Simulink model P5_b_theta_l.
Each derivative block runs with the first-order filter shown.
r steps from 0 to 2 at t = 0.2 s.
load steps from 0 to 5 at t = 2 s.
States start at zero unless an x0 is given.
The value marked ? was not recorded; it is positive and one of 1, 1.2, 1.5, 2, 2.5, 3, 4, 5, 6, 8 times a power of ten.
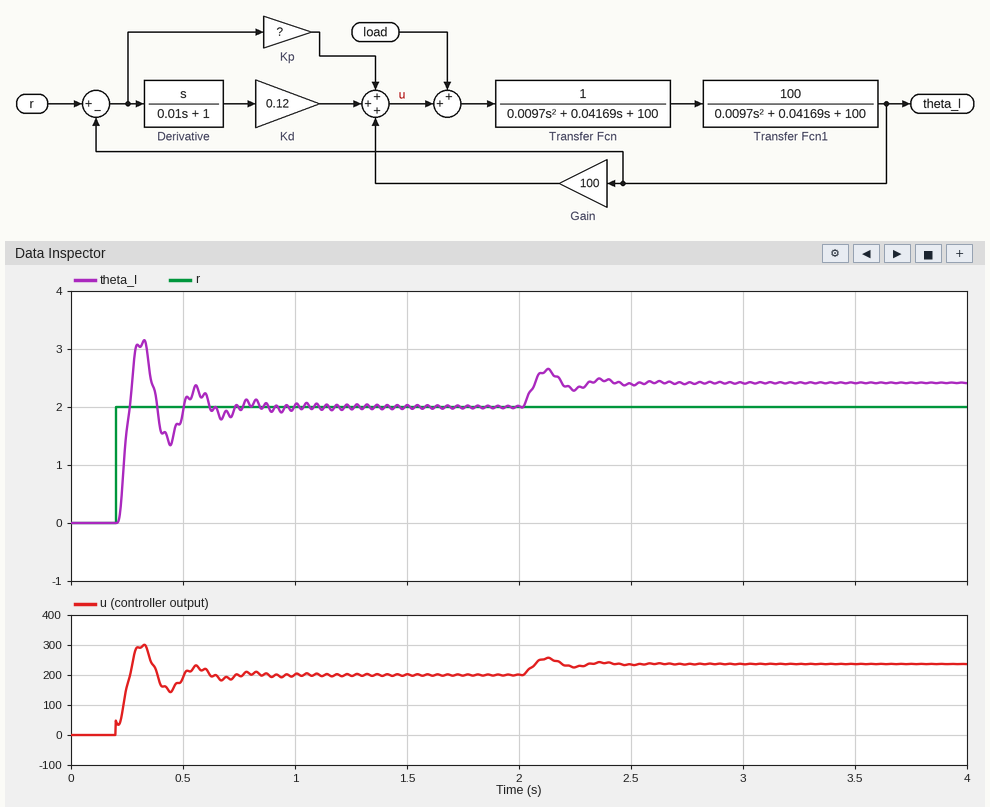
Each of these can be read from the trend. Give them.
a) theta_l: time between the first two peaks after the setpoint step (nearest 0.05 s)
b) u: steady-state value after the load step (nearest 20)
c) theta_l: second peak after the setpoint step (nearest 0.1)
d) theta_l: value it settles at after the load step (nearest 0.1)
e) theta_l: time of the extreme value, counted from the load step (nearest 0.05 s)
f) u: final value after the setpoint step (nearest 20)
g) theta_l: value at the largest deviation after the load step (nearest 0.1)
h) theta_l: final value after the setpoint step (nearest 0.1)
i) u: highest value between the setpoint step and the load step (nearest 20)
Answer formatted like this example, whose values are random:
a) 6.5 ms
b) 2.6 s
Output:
a) 0.25 s
b) 240
c) 2.4
d) 2.4
e) 0.15 s
f) 200
g) 2.7
h) 2.0
i) 300
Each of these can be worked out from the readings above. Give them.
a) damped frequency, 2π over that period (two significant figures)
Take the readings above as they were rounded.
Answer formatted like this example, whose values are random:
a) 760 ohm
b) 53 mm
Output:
a) 25 rad/s
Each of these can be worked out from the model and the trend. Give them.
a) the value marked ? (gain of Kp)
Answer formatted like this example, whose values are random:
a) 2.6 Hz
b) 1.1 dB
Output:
a) 12
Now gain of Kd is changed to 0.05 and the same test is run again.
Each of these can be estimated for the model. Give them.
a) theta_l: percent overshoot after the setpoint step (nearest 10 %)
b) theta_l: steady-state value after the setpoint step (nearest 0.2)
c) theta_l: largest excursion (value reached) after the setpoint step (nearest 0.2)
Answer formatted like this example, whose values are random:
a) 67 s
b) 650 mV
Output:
a) 70 %
b) 2.0
c) 3.4
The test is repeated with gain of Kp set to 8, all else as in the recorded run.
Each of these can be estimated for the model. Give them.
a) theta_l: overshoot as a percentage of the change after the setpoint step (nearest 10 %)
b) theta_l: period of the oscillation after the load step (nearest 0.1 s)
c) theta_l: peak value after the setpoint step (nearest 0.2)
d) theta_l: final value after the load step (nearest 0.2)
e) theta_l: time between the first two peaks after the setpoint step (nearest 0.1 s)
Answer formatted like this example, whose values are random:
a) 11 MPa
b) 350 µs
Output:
a) 50 %
b) 0.3 s
c) 3.0
d) 2.6
e) 0.3 s
